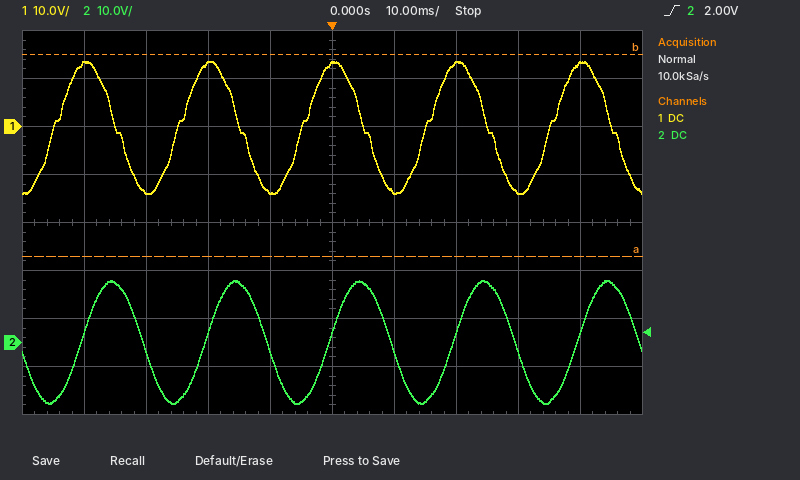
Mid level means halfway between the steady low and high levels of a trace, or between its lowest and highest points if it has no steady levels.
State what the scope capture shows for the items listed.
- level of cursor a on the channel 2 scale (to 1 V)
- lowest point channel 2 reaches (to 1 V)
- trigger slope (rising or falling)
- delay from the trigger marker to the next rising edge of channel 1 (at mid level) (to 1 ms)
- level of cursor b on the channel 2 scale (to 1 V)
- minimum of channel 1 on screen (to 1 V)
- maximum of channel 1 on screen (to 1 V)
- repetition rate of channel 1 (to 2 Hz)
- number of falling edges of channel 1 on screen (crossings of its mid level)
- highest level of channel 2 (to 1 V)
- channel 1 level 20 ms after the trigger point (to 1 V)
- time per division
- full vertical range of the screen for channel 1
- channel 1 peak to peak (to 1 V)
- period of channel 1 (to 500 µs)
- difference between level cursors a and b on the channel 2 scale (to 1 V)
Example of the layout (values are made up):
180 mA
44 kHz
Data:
18 V
-13 V
rising
15 ms
60 V
-14 V
14 V
50 Hz
5
13 V
13 V
10 ms
80 V
28 V
20.0 ms
42 V
